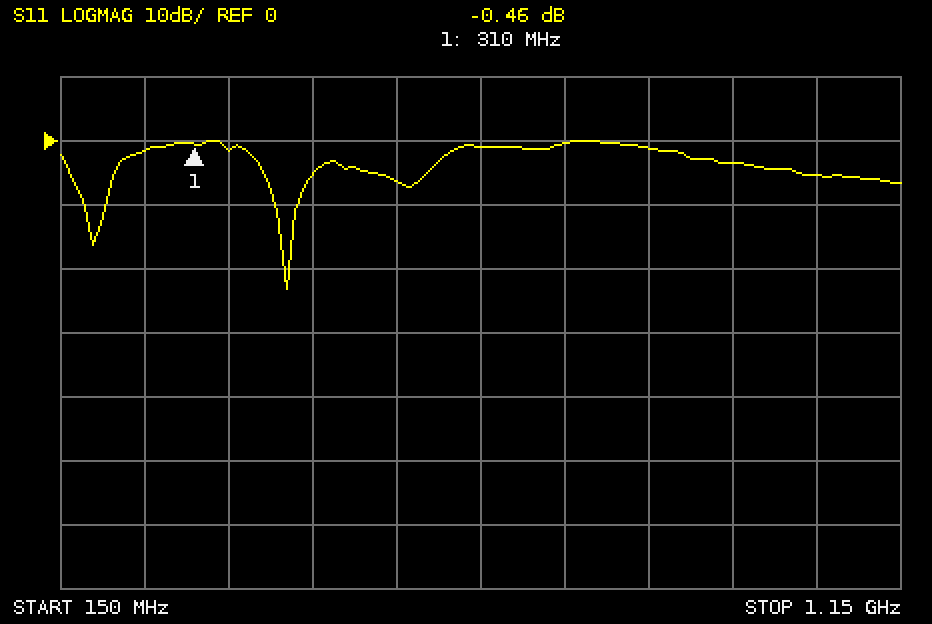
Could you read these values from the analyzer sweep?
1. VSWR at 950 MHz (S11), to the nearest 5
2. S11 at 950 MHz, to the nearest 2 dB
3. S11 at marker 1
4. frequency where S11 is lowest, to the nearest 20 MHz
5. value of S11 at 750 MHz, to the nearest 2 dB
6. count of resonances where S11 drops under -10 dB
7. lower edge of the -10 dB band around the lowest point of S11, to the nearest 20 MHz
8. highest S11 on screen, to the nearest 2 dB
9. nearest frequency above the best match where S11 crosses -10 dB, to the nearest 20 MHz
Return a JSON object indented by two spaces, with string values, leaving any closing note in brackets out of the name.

{
  "VSWR at 950 MHz (S11), to the nearest 5": "5",
  "S11 at 950 MHz, to the nearest 2 dB": "-4 dB",
  "S11 at marker 1": "-0.46 dB",
  "frequency where S11 is lowest, to the nearest 20 MHz": "420 MHz",
  "value of S11 at 750 MHz, to the nearest 2 dB": "0 dB",
  "count of resonances where S11 drops under -10 dB": "2",
  "lower edge of the -10 dB band around the lowest point of S11, to the nearest 20 MHz": "400 MHz",
  "highest S11 on screen, to the nearest 2 dB": "0 dB",
  "nearest frequency above the best match where S11 crosses -10 dB, to the nearest 20 MHz": "440 MHz"
}
